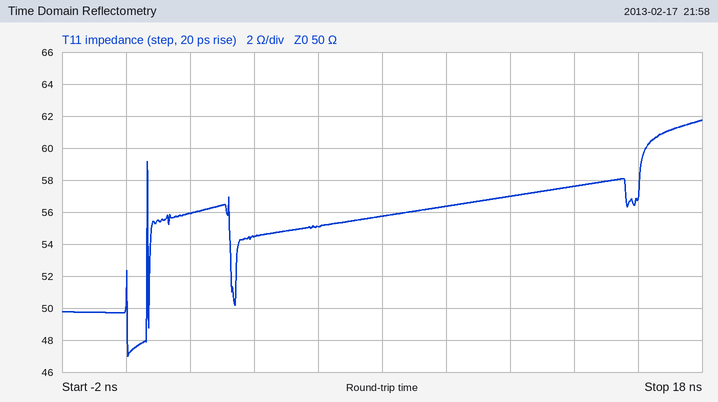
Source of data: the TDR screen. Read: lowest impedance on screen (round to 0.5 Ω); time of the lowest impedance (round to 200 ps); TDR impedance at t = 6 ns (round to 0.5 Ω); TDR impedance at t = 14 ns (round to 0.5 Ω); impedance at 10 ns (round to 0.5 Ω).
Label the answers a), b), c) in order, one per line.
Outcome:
a) 47.0 Ω
b) 0.0 ns
c) 55.0 Ω
d) 57.5 Ω
e) 56.5 Ω
